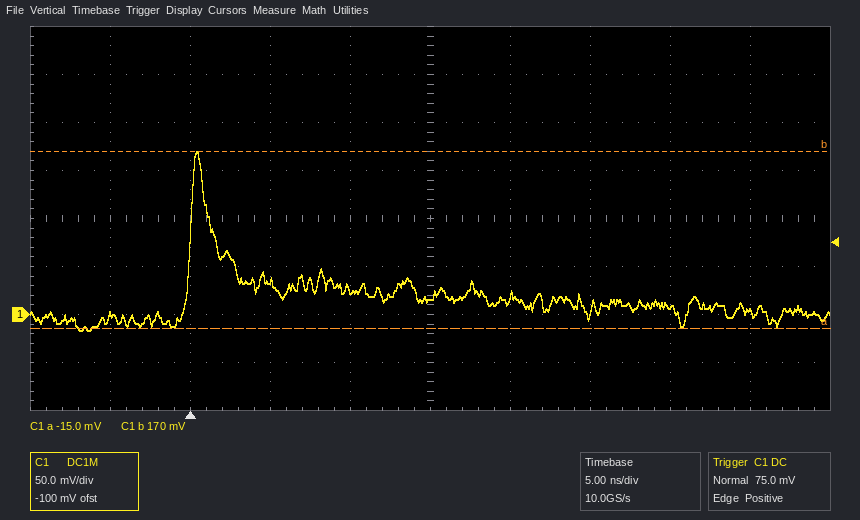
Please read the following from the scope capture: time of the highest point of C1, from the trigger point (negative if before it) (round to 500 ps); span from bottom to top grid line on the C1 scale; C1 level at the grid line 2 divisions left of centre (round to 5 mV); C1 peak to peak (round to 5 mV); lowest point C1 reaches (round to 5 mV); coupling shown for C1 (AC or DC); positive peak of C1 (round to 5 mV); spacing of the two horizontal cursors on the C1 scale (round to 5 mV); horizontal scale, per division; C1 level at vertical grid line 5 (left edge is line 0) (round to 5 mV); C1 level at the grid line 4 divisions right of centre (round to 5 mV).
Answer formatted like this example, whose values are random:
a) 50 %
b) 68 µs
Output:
a) +500 ps
b) 400 mV
c) 35 mV
d) 185 mV
e) -15 mV
f) DC
g) 170 mV
h) 185 mV
i) 5 ns
j) 15 mV
k) 0 mV
